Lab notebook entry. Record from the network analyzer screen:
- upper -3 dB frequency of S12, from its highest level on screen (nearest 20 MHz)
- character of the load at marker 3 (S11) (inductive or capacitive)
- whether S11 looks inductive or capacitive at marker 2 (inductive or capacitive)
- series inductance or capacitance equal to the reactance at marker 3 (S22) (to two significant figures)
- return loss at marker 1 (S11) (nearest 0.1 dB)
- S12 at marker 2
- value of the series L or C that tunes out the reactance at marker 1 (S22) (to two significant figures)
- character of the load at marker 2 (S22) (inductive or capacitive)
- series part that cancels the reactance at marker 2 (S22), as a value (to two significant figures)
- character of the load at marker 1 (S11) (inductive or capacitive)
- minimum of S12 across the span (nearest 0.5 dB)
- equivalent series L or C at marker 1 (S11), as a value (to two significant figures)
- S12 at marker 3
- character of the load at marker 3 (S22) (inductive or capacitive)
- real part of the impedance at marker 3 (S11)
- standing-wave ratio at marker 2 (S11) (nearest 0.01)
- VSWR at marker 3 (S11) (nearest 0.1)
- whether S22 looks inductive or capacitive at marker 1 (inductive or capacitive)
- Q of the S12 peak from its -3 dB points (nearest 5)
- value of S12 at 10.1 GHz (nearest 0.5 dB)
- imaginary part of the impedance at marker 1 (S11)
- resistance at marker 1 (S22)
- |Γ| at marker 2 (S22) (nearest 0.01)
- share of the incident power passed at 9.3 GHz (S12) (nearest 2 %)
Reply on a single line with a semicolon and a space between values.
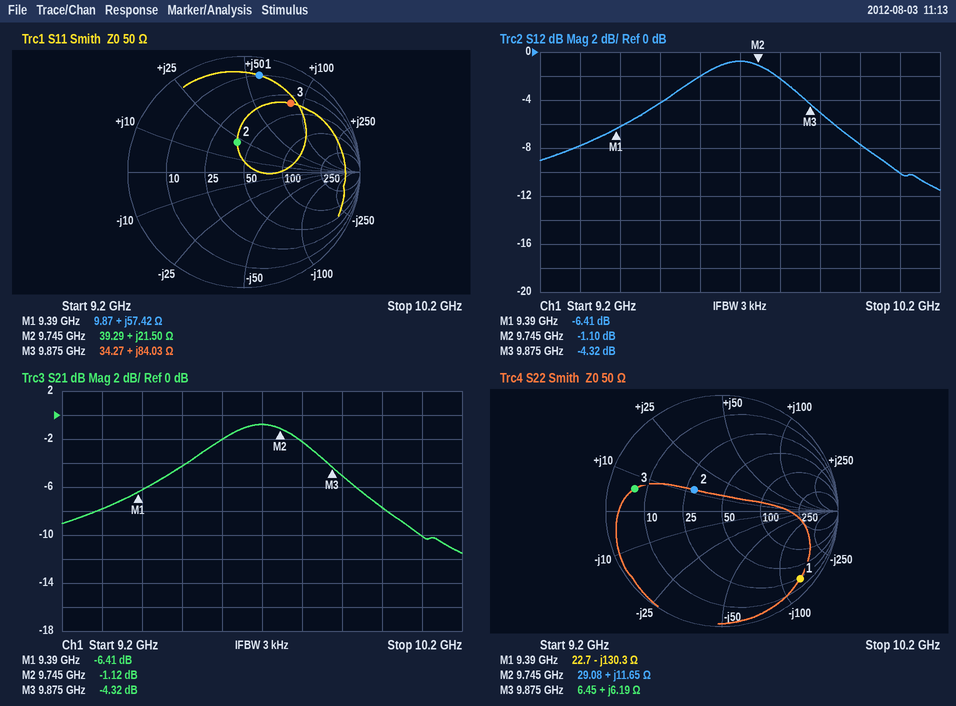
9.86 GHz; inductive; inductive; 100 pH; 1.5 dB; -1.10 dB; 2.2 nH; inductive; 1.4 pF; inductive; -11.5 dB; 970 pH; -4.32 dB; inductive; 34.27 Ω; 1.71; 6.1; capacitive; 30; -10.0 dB; +57.42 Ω; 22.7 Ω; 0.30; 16 %
